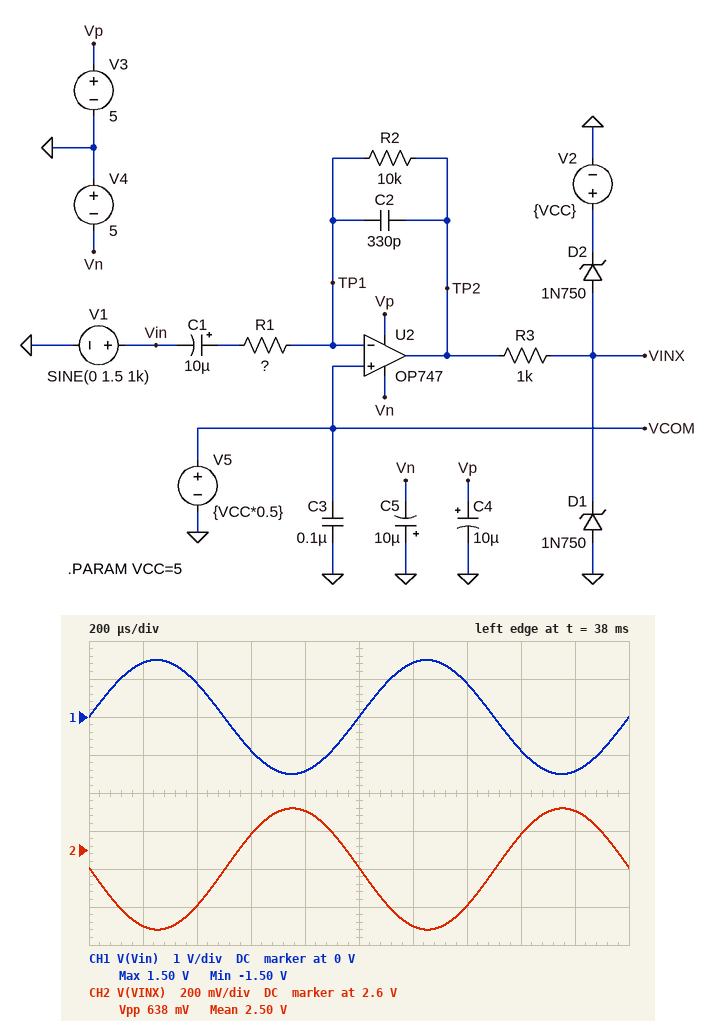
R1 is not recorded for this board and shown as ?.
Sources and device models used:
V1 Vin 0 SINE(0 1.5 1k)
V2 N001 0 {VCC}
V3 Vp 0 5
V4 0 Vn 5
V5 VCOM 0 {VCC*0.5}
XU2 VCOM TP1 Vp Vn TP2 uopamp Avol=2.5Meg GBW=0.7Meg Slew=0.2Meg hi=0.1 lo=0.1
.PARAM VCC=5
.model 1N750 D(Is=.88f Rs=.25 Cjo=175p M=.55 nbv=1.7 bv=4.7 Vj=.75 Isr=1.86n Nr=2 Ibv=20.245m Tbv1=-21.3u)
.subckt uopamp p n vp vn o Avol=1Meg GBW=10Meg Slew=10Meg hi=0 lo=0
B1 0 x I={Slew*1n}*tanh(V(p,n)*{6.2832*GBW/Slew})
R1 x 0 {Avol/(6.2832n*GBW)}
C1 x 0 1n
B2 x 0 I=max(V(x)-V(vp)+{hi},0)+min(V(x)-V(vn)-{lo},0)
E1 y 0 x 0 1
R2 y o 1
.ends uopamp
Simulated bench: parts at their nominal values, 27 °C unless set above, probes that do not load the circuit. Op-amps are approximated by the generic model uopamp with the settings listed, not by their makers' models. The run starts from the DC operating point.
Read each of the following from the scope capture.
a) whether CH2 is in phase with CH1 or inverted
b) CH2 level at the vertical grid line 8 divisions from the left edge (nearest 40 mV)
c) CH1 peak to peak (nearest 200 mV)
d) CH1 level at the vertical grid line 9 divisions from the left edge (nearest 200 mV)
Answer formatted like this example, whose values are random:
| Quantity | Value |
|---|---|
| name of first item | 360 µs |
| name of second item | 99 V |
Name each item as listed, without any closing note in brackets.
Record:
| Quantity | Value |
|---|---|
| whether CH2 is in phase with CH1 or inverted | inverted |
| CH2 level at the vertical grid line 8 divisions from the left edge | 2.68 V |
| CH1 peak to peak | 3.0 V |
| CH1 level at the vertical grid line 9 divisions from the left edge | -1.4 V |
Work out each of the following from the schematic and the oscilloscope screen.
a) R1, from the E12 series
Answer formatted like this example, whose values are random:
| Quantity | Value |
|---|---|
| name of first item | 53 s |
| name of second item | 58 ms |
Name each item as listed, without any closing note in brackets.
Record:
| Quantity | Value |
|---|---|
| R1, from the E12 series | 47 kΩ |
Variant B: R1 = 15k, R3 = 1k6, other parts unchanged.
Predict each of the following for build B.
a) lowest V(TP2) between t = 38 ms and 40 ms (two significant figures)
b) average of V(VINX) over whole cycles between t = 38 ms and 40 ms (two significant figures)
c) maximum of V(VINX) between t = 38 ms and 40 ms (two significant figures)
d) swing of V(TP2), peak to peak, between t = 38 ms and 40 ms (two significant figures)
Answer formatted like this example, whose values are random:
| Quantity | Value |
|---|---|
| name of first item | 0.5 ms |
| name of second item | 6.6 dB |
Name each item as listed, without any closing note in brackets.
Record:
| Quantity | Value |
|---|---|
| lowest V(TP2) between t = 38 ms and 40 ms | 1.5 V |
| average of V(VINX) over whole cycles between t = 38 ms and 40 ms | 2.5 V |
| maximum of V(VINX) between t = 38 ms and 40 ms | 3.5 V |
| swing of V(TP2), peak to peak, between t = 38 ms and 40 ms | 2.0 V |
